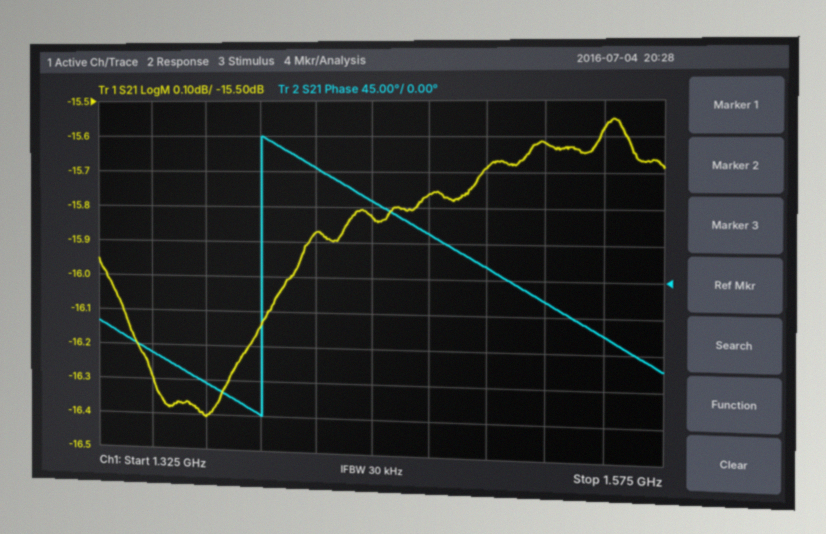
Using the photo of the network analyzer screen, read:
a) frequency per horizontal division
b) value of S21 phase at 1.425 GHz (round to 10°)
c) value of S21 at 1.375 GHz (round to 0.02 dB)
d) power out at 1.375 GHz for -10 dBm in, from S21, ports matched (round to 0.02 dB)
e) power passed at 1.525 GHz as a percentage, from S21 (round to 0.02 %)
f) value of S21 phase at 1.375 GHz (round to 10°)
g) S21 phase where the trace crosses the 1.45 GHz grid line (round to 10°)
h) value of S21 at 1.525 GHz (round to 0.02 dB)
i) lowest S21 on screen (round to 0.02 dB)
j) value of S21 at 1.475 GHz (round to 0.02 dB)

25 MHz
140°
-16.40 dB
-26.40 dBm
2.74 %
-140°
100°
-15.62 dB
-16.40 dB
-15.76 dB
